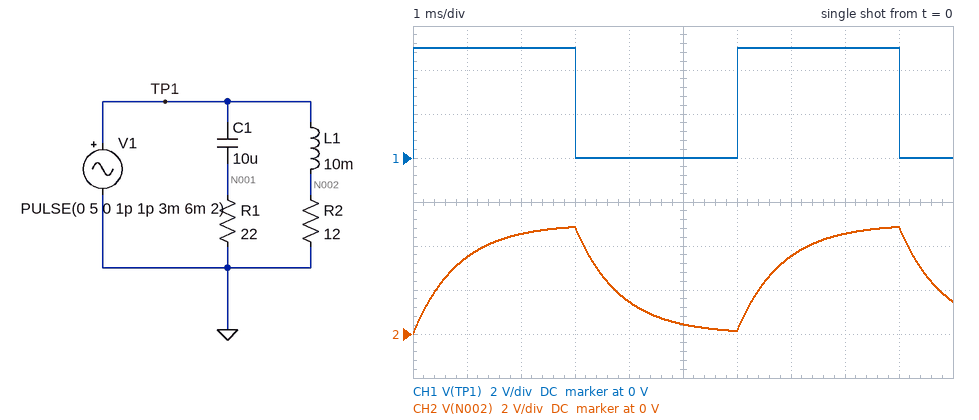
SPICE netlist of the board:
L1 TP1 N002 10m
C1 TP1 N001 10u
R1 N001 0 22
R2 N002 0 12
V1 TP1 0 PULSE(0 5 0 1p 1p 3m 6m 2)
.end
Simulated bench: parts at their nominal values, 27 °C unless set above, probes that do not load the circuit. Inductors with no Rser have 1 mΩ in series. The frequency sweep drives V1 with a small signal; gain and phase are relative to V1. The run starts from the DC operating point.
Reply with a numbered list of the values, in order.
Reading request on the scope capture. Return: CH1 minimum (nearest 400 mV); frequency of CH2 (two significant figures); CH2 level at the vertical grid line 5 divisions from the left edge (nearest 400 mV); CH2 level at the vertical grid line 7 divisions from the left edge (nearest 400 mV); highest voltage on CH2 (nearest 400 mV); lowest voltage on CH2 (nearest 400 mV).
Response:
1. 0 V
2. 170 Hz
3. 400 mV
4. 3.6 V
5. 4.8 V
6. 0 V
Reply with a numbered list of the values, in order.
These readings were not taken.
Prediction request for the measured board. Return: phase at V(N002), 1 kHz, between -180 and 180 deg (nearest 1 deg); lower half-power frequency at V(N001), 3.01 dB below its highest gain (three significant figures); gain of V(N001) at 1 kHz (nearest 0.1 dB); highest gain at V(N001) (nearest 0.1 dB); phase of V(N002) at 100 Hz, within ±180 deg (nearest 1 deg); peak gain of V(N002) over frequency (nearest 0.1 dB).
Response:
1. -79 deg
2. 723 Hz
3. -1.8 dB
4. 0 dB
5. -28 deg
6. 0 dB
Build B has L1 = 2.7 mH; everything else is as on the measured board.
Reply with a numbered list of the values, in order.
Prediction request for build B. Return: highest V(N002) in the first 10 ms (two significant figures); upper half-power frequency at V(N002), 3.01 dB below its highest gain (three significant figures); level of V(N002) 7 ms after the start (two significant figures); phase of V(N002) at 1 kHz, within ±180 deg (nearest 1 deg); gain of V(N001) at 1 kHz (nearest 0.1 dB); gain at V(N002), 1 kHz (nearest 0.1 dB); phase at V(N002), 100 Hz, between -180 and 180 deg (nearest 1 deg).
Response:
1. 5.0 V
2. 707 Hz
3. 4.9 V
4. -55 deg
5. -1.8 dB
6. -4.8 dB
7. -8 deg
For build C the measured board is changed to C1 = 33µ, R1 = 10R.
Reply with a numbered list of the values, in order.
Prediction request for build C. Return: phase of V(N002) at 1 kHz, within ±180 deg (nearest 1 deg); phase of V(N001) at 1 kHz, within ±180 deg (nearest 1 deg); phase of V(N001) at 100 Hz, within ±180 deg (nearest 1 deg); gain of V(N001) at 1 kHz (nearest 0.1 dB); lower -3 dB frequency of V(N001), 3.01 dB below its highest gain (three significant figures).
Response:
1. -79 deg
2. 26 deg
3. 78 deg
4. -0.9 dB
5. 482 Hz
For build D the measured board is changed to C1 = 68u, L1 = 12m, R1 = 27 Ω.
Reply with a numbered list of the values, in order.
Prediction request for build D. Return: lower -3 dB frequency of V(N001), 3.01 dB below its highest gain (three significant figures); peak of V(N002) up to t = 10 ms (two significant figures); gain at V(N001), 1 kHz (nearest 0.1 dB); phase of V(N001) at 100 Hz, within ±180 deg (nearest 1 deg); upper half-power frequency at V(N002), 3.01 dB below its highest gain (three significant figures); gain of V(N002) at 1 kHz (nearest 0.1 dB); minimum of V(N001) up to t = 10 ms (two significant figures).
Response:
1. 86.7 Hz
2. 4.8 V
3. 0 dB
4. 41 deg
5. 159 Hz
6. -16.1 dB
7. -4.2 V
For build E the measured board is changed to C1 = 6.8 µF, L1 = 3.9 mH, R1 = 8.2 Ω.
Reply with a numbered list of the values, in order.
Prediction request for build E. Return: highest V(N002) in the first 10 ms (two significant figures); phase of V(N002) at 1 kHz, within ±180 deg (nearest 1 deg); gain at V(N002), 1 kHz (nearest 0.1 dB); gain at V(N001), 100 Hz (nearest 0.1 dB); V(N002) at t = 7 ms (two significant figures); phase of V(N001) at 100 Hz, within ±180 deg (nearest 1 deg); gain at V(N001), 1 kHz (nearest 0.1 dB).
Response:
1. 5.0 V
2. -64 deg
3. -7.1 dB
4. -29.1 dB
5. 4.8 V
6. 88 deg
7. -9.6 dB
